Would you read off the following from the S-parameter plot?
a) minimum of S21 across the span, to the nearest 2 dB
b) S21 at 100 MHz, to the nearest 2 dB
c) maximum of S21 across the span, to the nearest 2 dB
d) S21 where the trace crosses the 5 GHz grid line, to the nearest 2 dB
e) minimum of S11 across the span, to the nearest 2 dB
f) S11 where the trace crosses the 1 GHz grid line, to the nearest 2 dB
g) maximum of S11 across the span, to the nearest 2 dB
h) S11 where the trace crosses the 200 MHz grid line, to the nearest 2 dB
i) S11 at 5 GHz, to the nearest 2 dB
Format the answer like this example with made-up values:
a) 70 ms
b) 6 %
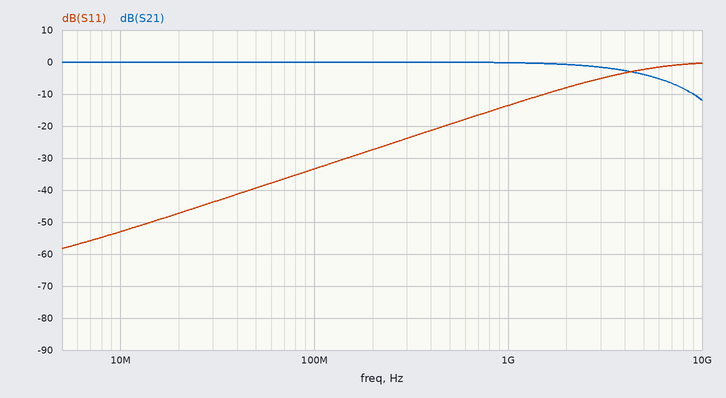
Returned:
a) -12 dB
b) 0 dB
c) 0 dB
d) -4 dB
e) -58 dB
f) -14 dB
g) 0 dB
h) -28 dB
i) -2 dB
